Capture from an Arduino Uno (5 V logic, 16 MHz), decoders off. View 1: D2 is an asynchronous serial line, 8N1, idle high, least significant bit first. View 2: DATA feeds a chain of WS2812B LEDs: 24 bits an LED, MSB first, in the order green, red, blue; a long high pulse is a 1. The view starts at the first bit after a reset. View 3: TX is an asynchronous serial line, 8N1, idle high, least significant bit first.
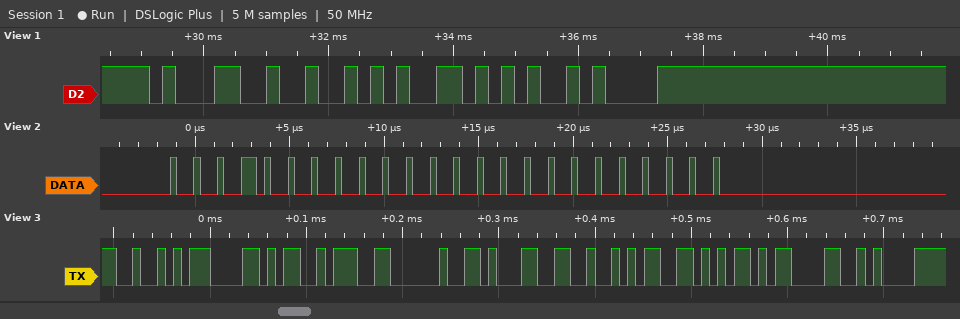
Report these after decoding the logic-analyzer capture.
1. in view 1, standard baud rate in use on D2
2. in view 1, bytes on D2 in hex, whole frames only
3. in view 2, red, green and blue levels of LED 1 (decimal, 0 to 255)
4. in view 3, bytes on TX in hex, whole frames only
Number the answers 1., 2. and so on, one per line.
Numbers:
1. 4800 baud
2. 31 52 56 0A
3. 0, 16, 0
4. 52 58 3A 20 31 52 56 0D 0A
